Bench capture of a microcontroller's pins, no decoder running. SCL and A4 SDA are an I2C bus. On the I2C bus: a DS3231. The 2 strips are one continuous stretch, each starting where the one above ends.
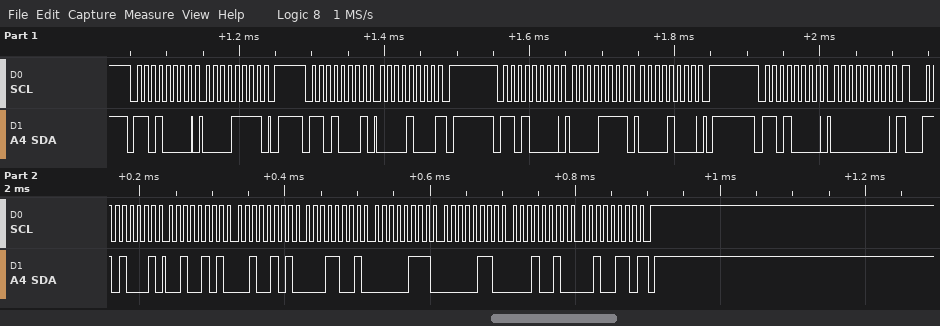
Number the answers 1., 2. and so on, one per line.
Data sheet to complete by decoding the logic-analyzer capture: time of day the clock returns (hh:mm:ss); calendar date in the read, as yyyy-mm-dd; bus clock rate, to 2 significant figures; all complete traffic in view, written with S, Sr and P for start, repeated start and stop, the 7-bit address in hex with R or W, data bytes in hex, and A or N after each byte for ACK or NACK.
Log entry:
1. 19:25:25
2. 2026-12-06
3. 100 kHz
4. S 68W A 0F A P S 68R A 08 N P S 68W A 0F A 08 A P S 68W A 00 A Sr 68R A 25 A 25 A 19 A 07 A 06 A 12 A 26 N P
